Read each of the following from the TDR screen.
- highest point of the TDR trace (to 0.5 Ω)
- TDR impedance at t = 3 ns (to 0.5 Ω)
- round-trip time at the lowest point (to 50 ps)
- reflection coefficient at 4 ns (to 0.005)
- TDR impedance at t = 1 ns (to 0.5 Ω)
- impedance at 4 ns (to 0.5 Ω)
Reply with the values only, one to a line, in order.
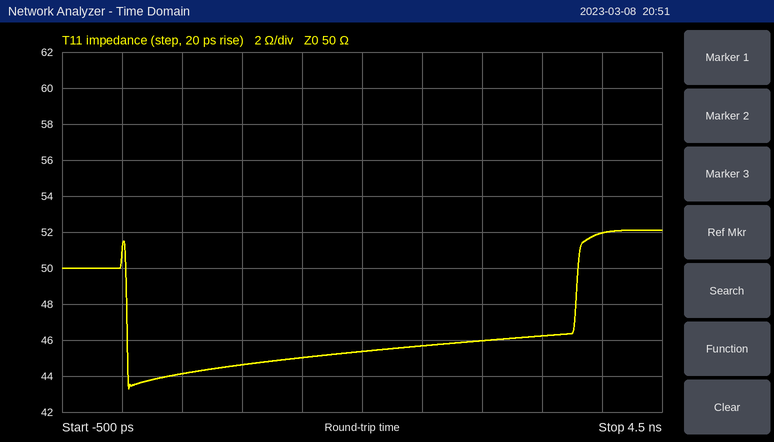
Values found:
52.0 Ω
46.0 Ω
50 ps
+0.020
44.5 Ω
52.0 Ω
